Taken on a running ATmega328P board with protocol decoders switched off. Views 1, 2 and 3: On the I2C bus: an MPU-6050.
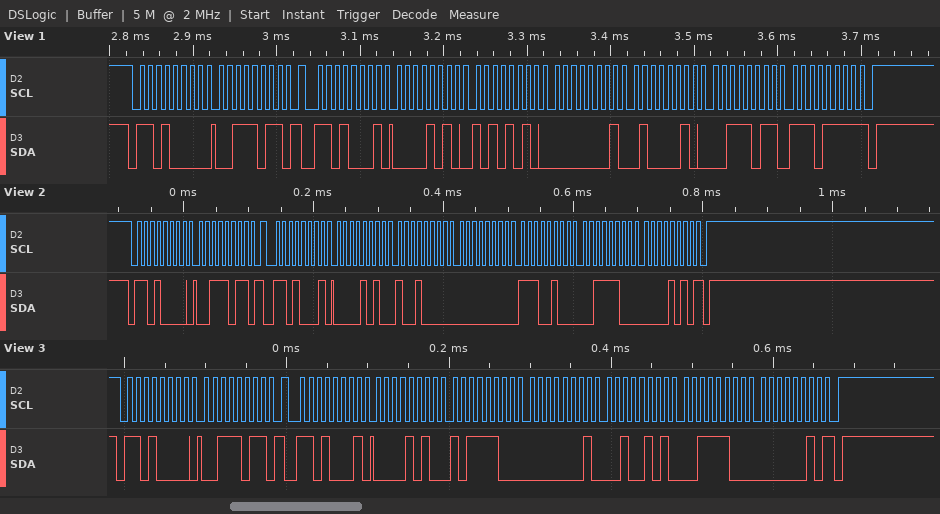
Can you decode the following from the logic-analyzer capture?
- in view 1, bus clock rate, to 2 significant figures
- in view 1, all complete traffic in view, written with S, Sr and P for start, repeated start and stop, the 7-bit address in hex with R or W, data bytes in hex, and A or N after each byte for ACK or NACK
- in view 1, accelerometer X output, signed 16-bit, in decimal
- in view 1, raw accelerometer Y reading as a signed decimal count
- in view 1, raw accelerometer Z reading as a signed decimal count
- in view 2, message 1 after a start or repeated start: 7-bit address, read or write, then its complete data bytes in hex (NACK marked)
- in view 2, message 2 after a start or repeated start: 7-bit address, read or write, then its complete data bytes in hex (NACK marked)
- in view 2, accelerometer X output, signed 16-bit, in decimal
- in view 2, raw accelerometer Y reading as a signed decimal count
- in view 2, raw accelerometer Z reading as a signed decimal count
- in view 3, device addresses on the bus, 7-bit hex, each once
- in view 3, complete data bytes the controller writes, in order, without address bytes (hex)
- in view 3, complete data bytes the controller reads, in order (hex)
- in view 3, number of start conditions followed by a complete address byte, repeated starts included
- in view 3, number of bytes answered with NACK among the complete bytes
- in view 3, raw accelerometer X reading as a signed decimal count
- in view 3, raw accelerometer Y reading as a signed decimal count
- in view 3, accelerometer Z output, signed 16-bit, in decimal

100 kHz
S 68W A 3B A Sr 68R A 0A A AA A 01 A 42 A 3B A EF N P
2730
322
15343
0x68 write: 3B
0x68 read: 0A 90 00 E4 3C 0A NACK
2704
228
15370
0x68
3B
0A BC 01 25 3C 02
2
1
2748
293
15362
